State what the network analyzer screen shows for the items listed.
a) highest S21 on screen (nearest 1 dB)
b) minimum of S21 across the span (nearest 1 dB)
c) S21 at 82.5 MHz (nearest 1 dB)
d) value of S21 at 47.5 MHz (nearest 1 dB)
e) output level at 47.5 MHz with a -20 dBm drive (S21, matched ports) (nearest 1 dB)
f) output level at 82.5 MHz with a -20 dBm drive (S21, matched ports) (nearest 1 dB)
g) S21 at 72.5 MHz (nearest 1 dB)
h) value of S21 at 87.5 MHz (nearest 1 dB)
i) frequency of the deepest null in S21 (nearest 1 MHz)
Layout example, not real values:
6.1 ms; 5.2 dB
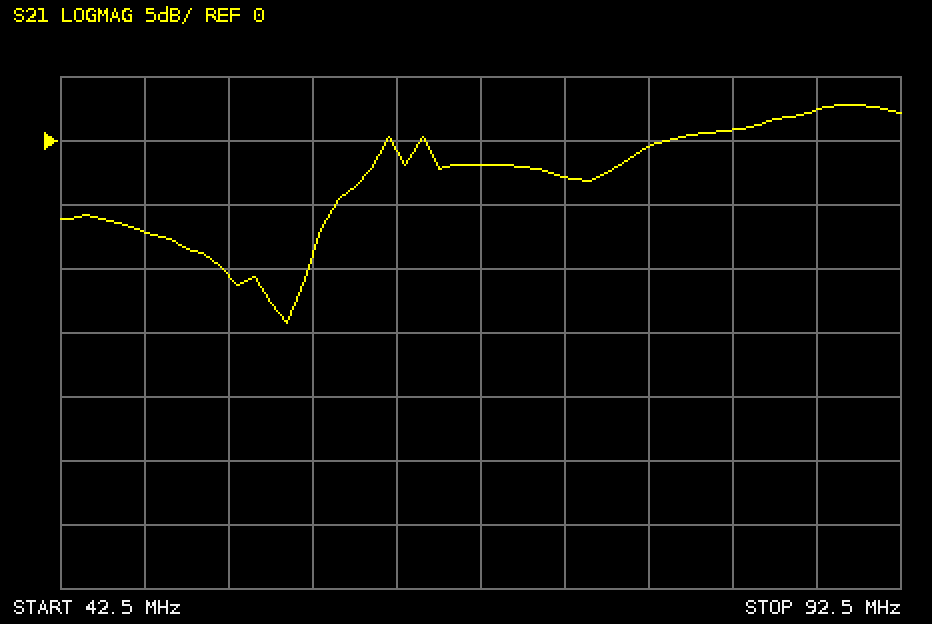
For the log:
3 dB; -14 dB; 1 dB; -7 dB; -27 dBm; -19 dBm; -3 dB; 2 dB; 56 MHz
